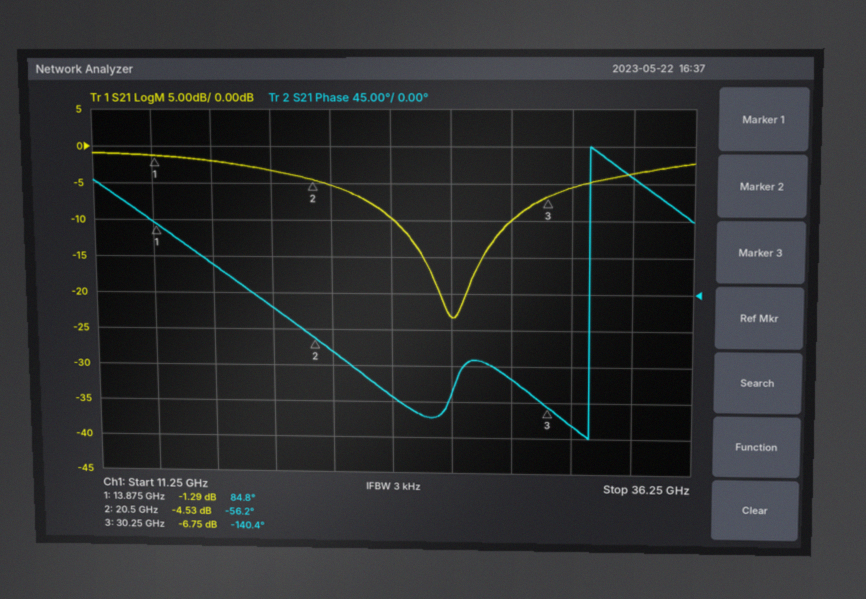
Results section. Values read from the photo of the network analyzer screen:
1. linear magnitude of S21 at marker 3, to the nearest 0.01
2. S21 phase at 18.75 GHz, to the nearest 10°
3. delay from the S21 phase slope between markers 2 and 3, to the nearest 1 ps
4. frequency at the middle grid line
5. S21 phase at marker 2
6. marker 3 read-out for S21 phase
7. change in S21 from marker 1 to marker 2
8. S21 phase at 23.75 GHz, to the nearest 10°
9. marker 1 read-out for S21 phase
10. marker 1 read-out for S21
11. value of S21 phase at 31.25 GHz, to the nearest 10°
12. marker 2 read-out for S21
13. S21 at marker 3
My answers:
0.46
-20°
24 ps
23.75 GHz
-56.2°
-140.4°
-3.24 dB
-130°
84.8°
-1.29 dB
-160°
-4.53 dB
-6.75 dB
